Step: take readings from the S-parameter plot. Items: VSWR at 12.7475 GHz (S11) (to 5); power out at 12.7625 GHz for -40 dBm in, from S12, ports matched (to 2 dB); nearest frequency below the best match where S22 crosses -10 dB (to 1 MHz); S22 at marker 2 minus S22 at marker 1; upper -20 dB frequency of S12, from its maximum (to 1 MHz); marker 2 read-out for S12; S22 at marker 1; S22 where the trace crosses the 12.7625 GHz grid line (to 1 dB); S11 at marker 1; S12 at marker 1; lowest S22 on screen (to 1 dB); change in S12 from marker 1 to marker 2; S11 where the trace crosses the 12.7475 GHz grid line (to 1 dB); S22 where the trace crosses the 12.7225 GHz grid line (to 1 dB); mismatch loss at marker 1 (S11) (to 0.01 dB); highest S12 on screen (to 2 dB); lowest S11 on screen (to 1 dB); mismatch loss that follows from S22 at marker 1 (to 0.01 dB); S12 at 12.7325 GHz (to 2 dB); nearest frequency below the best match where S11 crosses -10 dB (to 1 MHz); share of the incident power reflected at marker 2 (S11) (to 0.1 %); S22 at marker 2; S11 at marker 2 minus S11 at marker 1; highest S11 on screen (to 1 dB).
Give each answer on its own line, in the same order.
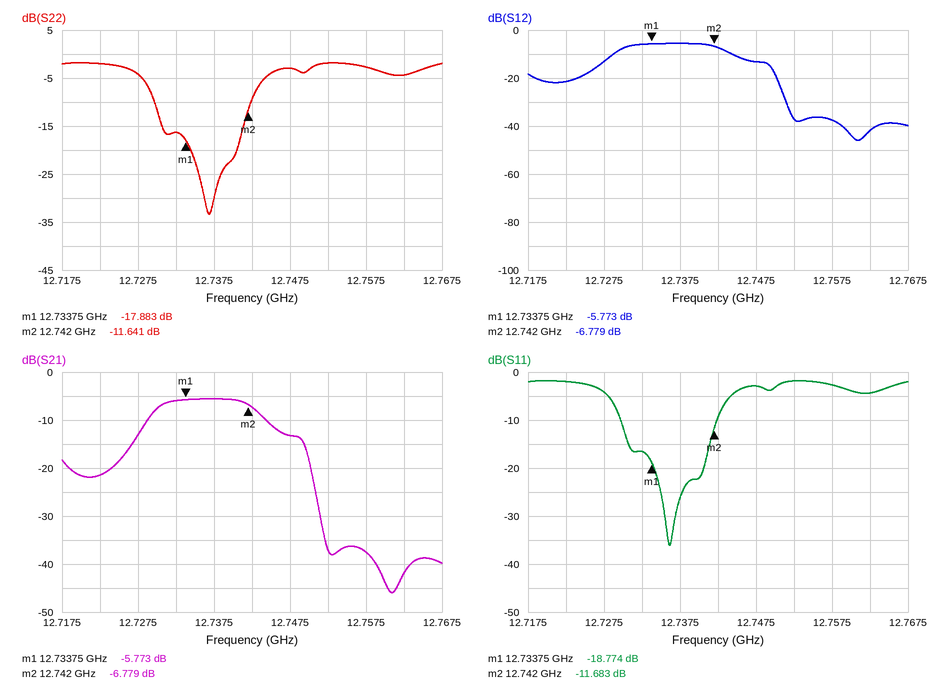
5
-82 dBm
12.730 GHz
6.242 dB
12.751 GHz
-6.779 dB
-17.883 dB
-4 dB
-18.774 dB
-5.773 dB
-33 dB
-1.006 dB
-3 dB
-2 dB
0.06 dB
-6 dB
-36 dB
0.07 dB
-6 dB
12.730 GHz
6.8 %
-11.641 dB
7.091 dB
-2 dB
